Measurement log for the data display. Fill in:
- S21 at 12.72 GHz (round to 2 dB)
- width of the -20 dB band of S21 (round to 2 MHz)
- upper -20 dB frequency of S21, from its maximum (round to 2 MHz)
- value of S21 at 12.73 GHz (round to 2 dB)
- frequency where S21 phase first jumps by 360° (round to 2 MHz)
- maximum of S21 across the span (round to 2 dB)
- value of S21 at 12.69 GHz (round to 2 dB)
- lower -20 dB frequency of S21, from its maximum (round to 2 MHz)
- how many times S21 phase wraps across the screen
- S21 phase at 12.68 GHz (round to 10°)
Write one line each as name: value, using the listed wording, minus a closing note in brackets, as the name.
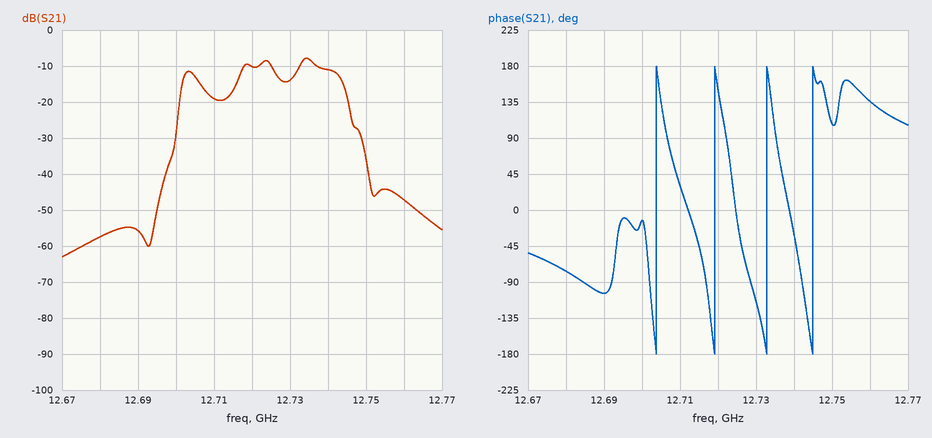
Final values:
S21 at 12.72 GHz: -10 dB
width of the -20 dB band of S21: 48 MHz
upper -20 dB frequency of S21, from its maximum: 12.748 GHz
value of S21 at 12.73 GHz: -14 dB
frequency where S21 phase first jumps by 360°: 12.704 GHz
maximum of S21 across the span: -8 dB
value of S21 at 12.69 GHz: -56 dB
lower -20 dB frequency of S21, from its maximum: 12.700 GHz
how many times S21 phase wraps across the screen: 4
S21 phase at 12.68 GHz: -80°
